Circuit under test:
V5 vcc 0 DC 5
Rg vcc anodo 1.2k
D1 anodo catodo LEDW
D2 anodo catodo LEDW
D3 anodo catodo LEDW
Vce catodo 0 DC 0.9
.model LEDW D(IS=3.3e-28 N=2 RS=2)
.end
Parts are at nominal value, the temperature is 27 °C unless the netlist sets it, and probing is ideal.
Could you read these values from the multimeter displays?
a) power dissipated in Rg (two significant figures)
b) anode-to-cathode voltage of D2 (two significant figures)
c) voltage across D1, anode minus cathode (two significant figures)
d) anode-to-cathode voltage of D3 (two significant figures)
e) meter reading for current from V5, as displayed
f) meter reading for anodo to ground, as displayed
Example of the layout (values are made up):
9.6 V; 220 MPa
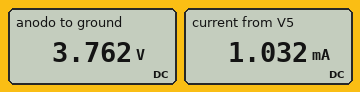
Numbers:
1.3 mW; 2.9 V; 2.9 V; 2.9 V; 1.032 mA; 3.762 V
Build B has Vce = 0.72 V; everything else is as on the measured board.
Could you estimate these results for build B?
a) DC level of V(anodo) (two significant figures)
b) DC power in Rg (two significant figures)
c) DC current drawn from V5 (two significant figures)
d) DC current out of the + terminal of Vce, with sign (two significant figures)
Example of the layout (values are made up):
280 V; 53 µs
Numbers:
3.6 V; 1.7 mW; 1.2 mA; -1.2 mA
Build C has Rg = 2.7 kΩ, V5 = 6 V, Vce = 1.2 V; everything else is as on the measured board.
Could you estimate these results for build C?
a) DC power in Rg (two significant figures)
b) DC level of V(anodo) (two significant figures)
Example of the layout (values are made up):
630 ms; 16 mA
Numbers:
1.4 mW; 4.0 V
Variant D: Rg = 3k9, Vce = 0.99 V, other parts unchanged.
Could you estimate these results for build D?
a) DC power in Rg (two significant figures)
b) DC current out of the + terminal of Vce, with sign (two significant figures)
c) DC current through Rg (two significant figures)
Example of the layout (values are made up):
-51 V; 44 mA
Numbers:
380 µW; -310 µA; 310 µA
